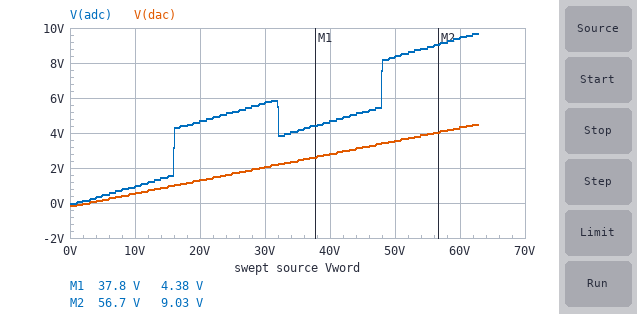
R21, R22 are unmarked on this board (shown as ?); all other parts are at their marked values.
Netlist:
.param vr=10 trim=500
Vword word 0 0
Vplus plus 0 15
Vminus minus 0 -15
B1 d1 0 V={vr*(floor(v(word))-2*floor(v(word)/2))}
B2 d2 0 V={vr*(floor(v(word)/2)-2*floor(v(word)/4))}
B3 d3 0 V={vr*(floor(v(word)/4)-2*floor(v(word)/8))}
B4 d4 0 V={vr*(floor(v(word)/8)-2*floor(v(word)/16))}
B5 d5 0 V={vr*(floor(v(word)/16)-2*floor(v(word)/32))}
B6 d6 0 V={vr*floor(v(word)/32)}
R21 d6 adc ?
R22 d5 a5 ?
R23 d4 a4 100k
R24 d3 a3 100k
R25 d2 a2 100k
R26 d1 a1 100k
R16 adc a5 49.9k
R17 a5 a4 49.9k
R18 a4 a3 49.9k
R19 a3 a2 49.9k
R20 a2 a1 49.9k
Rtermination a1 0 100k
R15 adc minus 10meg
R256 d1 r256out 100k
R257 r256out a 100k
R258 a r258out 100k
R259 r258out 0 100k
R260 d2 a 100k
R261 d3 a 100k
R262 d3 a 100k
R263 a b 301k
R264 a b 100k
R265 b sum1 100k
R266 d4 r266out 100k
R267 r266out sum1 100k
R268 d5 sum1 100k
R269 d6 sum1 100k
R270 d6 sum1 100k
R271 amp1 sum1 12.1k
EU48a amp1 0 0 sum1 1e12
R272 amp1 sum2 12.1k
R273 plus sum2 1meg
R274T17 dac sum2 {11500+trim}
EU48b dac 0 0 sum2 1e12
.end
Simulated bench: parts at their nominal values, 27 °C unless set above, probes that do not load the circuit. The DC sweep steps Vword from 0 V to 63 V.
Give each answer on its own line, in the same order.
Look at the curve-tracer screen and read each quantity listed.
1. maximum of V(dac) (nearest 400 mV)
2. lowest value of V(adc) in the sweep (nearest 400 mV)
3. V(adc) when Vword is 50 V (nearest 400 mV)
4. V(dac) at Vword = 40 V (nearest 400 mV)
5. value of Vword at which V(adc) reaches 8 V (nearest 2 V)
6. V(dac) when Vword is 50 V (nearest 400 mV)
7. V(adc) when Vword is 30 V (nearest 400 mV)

4.4 V
0 V
8.4 V
2.8 V
48 V
3.6 V
5.6 V
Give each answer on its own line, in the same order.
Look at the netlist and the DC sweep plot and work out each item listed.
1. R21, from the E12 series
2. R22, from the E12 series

120 kΩ
39 kΩ
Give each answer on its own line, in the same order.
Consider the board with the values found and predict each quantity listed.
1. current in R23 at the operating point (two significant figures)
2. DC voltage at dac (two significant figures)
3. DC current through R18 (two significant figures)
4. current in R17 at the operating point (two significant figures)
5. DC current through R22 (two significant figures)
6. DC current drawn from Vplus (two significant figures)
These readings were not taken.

130 nA
-180 mV
130 nA
250 nA
650 nA
15 µA
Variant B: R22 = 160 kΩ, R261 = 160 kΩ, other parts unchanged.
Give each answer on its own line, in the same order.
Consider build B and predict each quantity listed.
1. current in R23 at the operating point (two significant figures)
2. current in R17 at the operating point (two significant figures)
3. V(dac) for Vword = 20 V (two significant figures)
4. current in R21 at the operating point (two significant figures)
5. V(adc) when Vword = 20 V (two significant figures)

240 nA
480 nA
1.3 V
720 nA
2.7 V
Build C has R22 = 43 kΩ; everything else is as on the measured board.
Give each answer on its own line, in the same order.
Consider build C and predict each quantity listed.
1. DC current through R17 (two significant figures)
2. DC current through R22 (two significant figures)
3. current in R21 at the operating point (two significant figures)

270 nA
630 nA
600 nA
